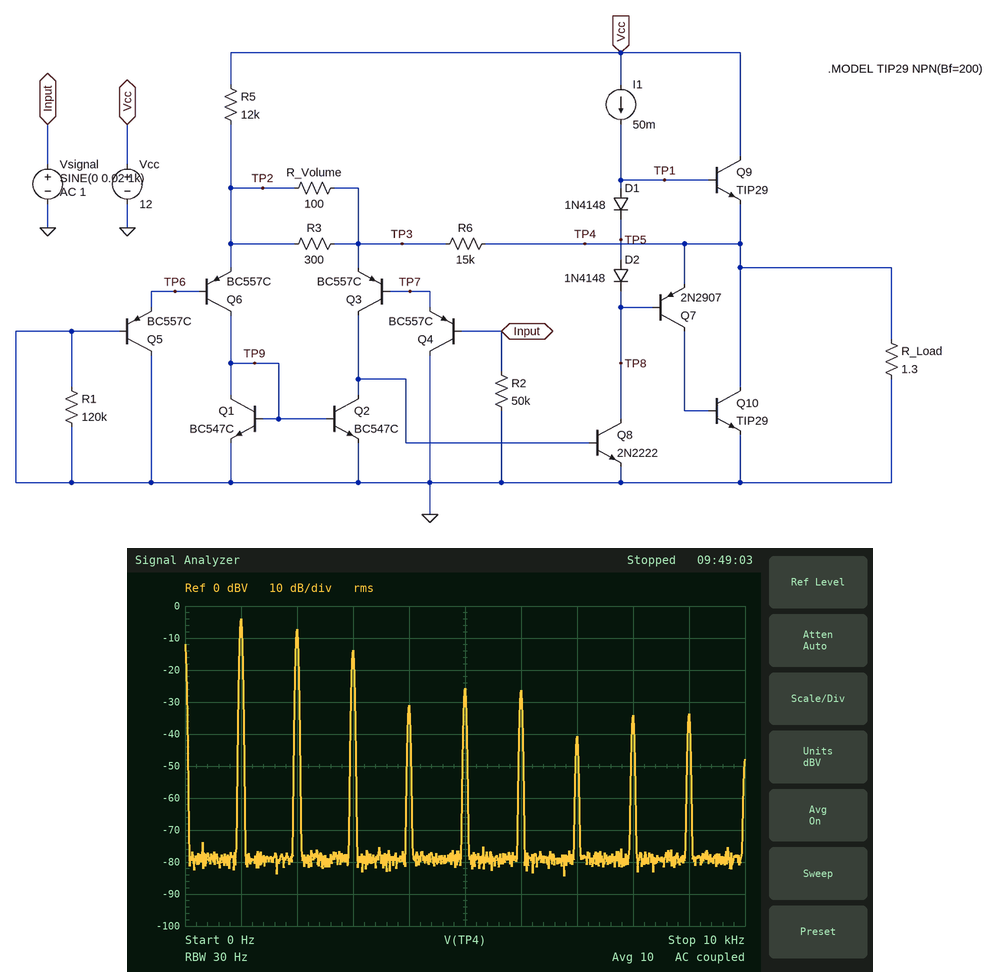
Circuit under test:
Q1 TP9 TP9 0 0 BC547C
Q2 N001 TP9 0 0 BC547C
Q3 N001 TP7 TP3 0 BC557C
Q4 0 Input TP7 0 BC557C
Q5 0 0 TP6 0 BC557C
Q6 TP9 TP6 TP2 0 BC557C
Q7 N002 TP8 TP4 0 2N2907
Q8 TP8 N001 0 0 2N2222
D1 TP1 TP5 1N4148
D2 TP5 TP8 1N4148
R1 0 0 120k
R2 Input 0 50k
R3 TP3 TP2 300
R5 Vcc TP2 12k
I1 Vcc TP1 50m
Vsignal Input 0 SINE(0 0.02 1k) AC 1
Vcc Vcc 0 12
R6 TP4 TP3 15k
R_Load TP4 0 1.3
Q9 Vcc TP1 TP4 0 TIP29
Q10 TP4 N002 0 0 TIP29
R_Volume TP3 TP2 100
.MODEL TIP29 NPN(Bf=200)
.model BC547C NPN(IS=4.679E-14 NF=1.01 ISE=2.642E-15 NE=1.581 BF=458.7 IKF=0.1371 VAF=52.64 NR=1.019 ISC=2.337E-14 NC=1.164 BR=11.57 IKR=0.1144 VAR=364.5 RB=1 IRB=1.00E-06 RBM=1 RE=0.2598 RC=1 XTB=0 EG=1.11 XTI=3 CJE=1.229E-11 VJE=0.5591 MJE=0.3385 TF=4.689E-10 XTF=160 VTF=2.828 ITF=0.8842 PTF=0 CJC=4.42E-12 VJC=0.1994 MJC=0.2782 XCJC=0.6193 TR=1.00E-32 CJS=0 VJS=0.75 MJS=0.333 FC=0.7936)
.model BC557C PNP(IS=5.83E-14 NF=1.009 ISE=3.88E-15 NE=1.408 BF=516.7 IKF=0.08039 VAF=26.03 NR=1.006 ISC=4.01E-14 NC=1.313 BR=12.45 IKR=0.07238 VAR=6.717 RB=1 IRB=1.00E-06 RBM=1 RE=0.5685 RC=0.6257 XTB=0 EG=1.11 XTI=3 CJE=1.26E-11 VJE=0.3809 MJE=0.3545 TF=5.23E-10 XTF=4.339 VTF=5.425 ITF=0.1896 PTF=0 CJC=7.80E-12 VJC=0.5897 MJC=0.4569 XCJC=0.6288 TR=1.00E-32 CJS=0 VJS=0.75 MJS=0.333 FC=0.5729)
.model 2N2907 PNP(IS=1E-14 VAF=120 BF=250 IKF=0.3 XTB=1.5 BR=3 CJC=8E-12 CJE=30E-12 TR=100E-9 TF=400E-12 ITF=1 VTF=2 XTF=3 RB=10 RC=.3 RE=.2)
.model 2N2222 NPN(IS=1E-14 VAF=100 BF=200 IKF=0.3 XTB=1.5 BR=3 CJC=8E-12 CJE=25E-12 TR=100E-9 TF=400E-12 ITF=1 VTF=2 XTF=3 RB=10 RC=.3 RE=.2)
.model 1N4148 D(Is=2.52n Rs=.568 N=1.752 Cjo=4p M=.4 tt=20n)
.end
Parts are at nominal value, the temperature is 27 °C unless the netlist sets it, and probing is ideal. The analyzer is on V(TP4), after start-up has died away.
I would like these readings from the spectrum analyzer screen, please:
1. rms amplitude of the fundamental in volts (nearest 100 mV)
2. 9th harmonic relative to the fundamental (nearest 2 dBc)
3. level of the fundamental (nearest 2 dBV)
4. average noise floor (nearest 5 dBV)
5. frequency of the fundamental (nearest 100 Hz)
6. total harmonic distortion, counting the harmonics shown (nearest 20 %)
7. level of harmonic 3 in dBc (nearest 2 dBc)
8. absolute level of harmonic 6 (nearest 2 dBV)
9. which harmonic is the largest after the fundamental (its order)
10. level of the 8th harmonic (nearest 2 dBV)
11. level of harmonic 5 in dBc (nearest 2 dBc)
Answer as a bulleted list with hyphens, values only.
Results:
- 600 mV
- -30 dBc
- -4 dBV
- -80 dBV
- 1.0 kHz
- 80 %
- -10 dBc
- -26 dBV
- 2
- -34 dBV
- -22 dBc
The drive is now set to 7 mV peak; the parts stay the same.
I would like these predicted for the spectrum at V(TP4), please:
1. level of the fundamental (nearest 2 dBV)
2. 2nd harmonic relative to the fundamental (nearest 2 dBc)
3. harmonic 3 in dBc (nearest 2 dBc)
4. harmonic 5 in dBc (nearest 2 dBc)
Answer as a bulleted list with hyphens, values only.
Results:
- -90 dBV
- 0 dBc
- 0 dBc
- -2 dBc
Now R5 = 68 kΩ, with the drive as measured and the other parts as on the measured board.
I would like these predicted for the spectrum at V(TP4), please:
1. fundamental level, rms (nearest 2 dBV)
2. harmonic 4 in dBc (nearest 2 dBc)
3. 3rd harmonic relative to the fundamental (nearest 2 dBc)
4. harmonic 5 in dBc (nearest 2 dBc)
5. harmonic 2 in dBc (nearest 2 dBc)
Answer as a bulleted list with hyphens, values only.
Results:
- 6 dBV
- -32 dBc
- -30 dBc
- -34 dBc
- -26 dBc
